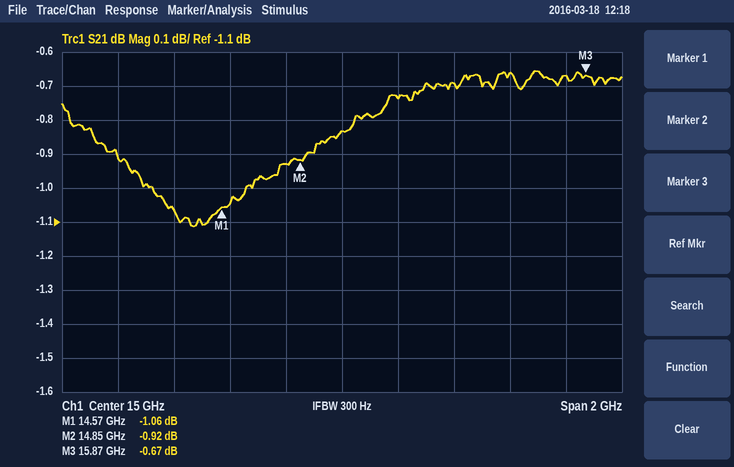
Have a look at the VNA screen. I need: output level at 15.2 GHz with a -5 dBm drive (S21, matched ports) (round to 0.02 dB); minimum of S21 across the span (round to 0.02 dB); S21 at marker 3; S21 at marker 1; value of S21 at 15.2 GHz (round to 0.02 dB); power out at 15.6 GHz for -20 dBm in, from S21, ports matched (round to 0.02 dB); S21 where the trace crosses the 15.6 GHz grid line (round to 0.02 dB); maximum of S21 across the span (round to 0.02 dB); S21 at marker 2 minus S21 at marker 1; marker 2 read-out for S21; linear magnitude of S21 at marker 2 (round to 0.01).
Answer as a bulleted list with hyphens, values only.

- -5.74 dBm
- -1.12 dB
- -0.67 dB
- -1.06 dB
- -0.74 dB
- -20.66 dBm
- -0.66 dB
- -0.66 dB
- 0.14 dB
- -0.92 dB
- 0.90
